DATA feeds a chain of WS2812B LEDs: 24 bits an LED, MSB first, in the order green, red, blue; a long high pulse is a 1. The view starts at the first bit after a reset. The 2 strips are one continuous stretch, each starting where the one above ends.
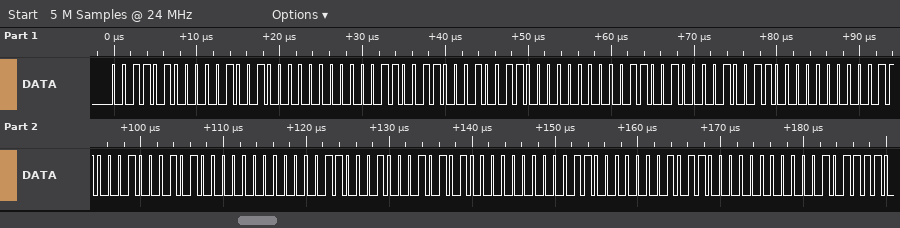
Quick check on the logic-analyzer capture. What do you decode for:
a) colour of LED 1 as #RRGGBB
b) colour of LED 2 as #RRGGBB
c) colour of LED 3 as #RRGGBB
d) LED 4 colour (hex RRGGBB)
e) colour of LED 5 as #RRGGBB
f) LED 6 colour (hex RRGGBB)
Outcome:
#123400
#133300
#133200
#143100
#153100
#163000
